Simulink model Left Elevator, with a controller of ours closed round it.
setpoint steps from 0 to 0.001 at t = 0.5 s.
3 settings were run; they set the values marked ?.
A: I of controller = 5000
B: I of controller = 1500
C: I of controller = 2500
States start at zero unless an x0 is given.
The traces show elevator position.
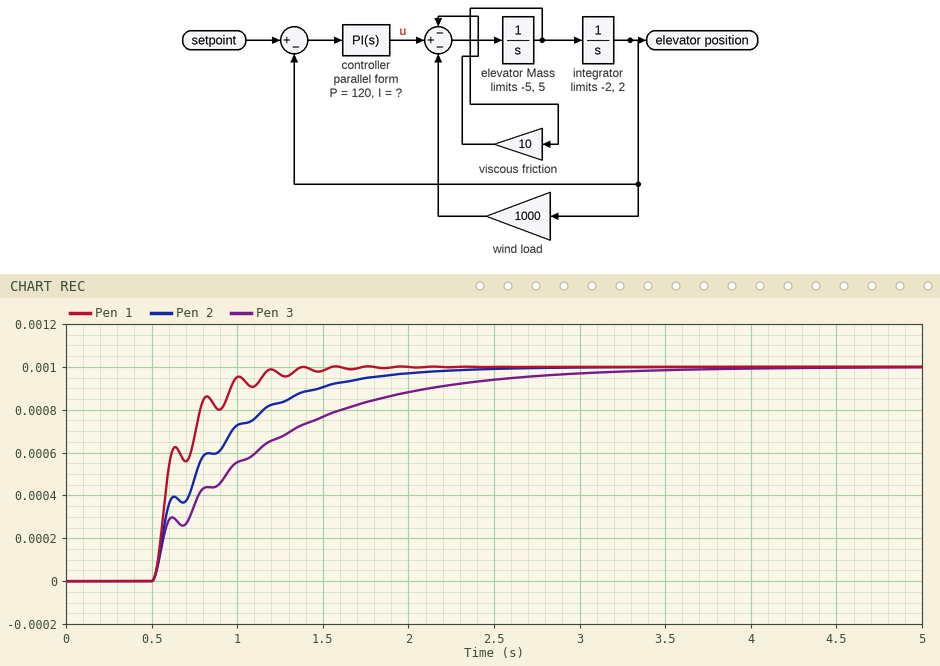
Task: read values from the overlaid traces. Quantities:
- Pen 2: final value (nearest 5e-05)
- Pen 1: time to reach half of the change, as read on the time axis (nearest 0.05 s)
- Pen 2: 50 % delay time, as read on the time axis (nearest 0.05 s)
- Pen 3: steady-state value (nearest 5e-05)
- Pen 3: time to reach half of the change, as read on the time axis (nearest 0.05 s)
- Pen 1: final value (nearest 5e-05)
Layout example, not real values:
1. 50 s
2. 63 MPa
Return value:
1. 0.00100
2. 0.60 s
3. 0.75 s
4. 0.00100
5. 0.95 s
6. 0.00100
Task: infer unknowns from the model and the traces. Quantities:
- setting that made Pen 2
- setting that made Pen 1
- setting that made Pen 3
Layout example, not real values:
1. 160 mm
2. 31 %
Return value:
1. C
2. A
3. B
